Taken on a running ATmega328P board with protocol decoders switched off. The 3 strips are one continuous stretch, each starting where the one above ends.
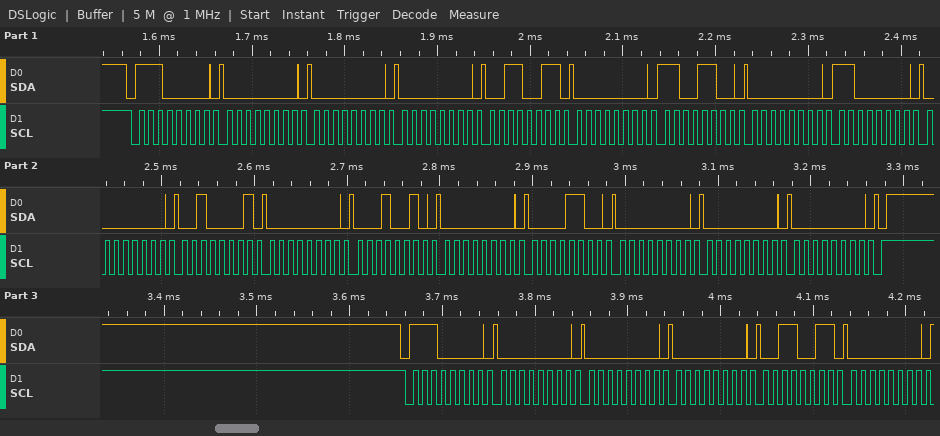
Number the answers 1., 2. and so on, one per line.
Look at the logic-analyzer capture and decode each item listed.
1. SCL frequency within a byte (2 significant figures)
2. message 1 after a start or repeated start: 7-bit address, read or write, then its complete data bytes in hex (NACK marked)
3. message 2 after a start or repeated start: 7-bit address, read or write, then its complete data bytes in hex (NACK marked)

1. 100 kHz
2. 0x70 write: 00 00 00 33 00 CC 00 C0 00 21 00 12 00 0C 00 00 00
3. 0x70 write: 00 00 00 33 00
